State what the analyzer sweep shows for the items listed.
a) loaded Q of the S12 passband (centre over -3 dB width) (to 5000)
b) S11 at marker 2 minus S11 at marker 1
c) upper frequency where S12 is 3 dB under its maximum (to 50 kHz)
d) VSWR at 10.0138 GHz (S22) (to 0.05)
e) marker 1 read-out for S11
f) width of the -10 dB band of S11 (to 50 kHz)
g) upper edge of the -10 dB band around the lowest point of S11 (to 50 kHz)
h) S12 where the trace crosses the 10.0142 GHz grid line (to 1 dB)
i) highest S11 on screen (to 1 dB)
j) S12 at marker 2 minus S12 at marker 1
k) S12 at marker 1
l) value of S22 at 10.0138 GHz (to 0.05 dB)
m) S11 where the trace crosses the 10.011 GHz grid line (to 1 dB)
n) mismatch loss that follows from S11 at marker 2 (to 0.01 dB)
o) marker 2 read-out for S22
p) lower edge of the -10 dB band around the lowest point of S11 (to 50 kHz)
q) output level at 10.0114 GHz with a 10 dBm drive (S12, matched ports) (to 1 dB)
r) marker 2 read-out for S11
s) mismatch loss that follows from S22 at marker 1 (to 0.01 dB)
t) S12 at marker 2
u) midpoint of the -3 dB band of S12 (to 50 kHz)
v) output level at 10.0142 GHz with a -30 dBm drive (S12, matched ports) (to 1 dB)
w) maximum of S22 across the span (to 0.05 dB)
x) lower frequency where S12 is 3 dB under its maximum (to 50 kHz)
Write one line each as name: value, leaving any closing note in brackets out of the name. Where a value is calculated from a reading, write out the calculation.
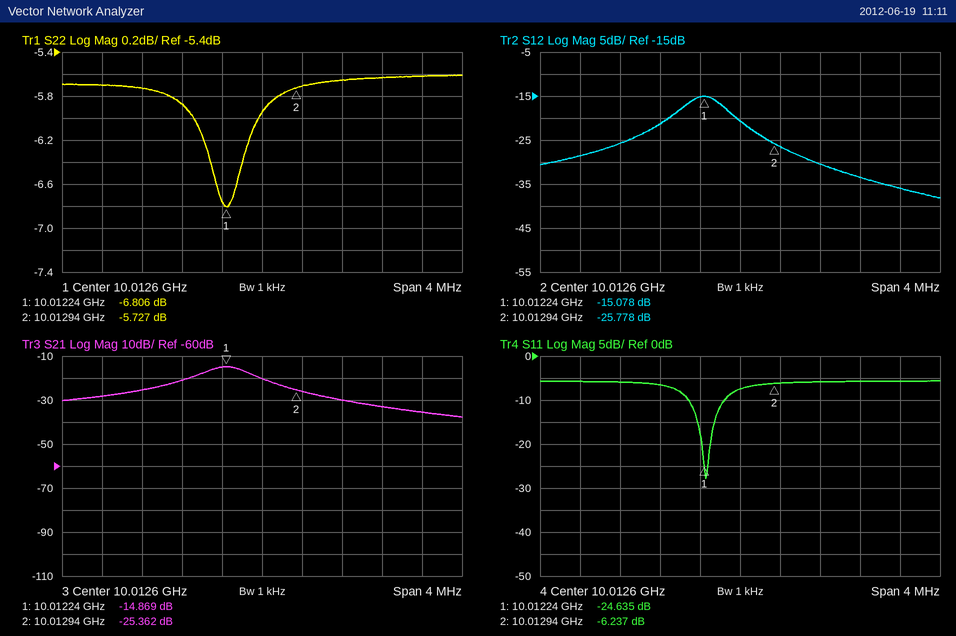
loaded Q of the S12 passband (centre over -3 dB width): 10.0122 GHz / 450 kHz ≈ 22249, so 20000 to the nearest 5000
S11 at marker 2 minus S11 at marker 1: -6.237 − (-24.635) = 18.398 dB
upper frequency where S12 is 3 dB under its maximum: 10.01245 GHz
VSWR at 10.0138 GHz (S22): |Γ| = 10^(-5.65/20) = 0.5218; VSWR = (1 + 0.5218)/(1 − 0.5218) ≈ 3.18, so 3.20 to the nearest 0.05
marker 1 read-out for S11: -24.635 dB
width of the -10 dB band of S11: 10.01245 GHz − 10.01210 GHz = 350 kHz
upper edge of the -10 dB band around the lowest point of S11: 10.01245 GHz
S12 where the trace crosses the 10.0142 GHz grid line: -36 dB
highest S11 on screen: -6 dB
S12 at marker 2 minus S12 at marker 1: -25.778 − (-15.078) = -10.700 dB
S12 at marker 1: -15.078 dB
value of S22 at 10.0138 GHz: -5.65 dB
S11 where the trace crosses the 10.011 GHz grid line: -6 dB
mismatch loss that follows from S11 at marker 2: −10 log10(1 − 10^(-6.237/10)) ≈ 1.18 dB
marker 2 read-out for S22: -5.727 dB
lower edge of the -10 dB band around the lowest point of S11: 10.01210 GHz
output level at 10.0114 GHz with a 10 dBm drive (S12, matched ports): 10 dBm + (-26 dB) = -16 dBm
marker 2 read-out for S11: -6.237 dB
mismatch loss that follows from S22 at marker 1: −10 log10(1 − 10^(-6.806/10)) ≈ 1.02 dB
S12 at marker 2: -25.778 dB
midpoint of the -3 dB band of S12: 10.01225 GHz
output level at 10.0142 GHz with a -30 dBm drive (S12, matched ports): -30 dBm + (-36 dB) = -66 dBm
maximum of S22 across the span: -5.60 dB
lower frequency where S12 is 3 dB under its maximum: 10.01200 GHz
